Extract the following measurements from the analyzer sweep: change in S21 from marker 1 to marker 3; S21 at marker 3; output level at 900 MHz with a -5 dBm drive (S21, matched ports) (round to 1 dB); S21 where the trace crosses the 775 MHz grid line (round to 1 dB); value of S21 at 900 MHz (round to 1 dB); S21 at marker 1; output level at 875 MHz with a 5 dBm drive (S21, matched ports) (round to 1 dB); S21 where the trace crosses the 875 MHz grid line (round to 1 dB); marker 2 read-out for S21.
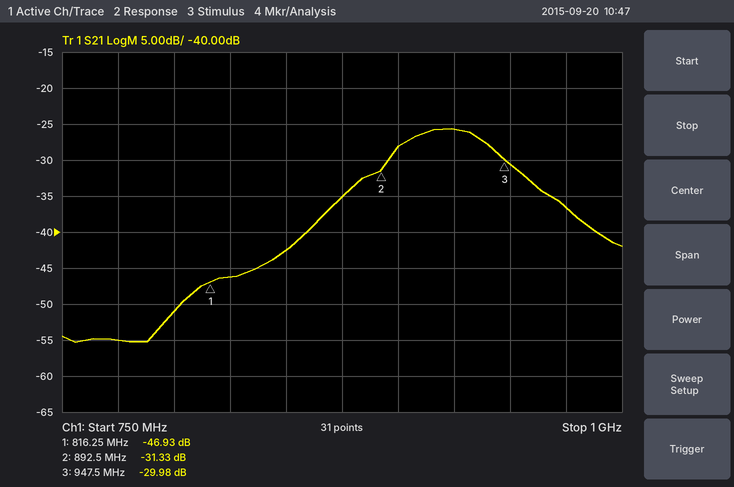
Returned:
16.95 dB
-29.98 dB
-33 dBm
-55 dB
-28 dB
-46.93 dB
-30 dBm
-35 dB
-31.33 dB
